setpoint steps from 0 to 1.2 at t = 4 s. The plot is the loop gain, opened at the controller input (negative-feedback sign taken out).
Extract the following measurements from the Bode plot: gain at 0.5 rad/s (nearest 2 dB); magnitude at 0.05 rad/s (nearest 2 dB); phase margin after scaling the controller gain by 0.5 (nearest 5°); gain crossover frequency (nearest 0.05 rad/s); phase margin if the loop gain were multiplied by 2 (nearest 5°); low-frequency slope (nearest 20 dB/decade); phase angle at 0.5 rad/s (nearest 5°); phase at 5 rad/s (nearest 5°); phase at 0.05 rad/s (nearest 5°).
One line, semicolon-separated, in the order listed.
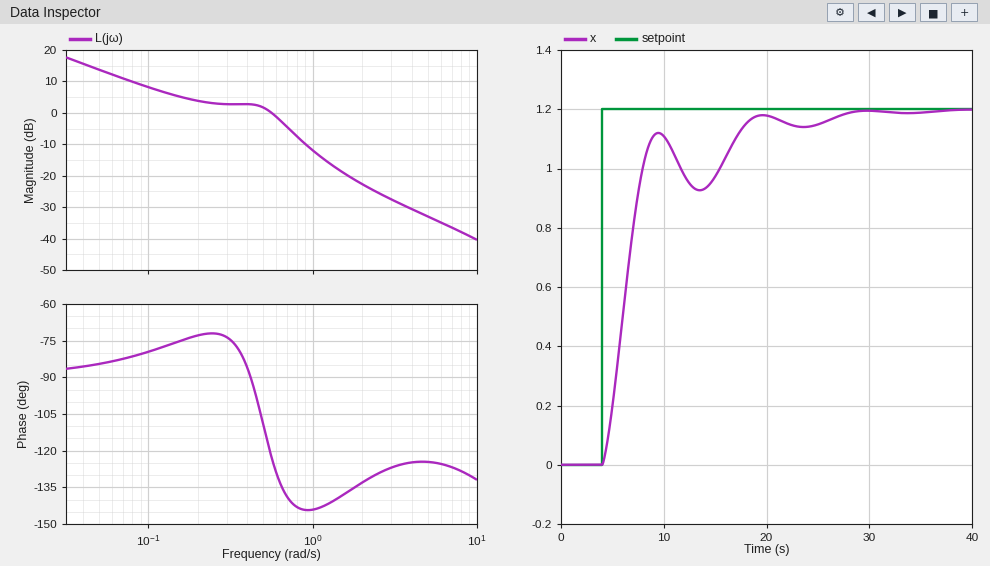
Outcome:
2 dB; 14 dB; 105°; 0.55 rad/s; 40°; -20 dB/decade; -110°; -125°; -85°
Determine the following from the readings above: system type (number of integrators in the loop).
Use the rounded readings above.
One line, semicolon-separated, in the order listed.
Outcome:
1
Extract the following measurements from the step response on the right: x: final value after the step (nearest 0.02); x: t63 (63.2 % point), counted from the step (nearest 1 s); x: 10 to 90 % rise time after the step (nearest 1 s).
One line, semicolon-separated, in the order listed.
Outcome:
1.20; 3 s; 4 s
